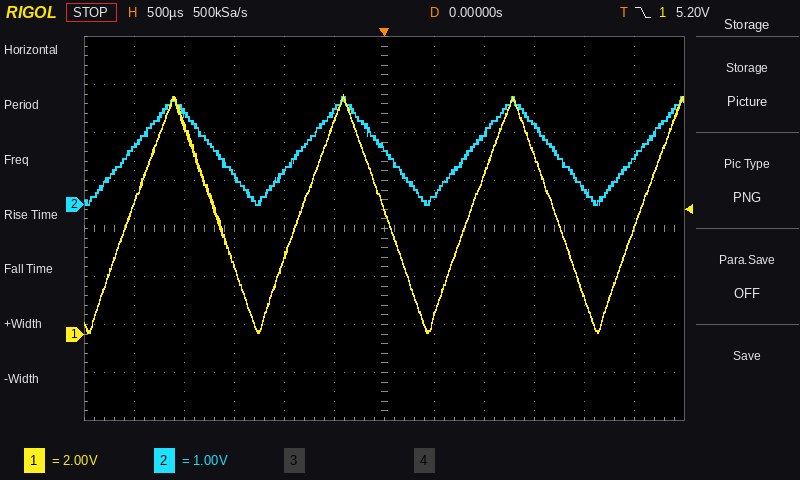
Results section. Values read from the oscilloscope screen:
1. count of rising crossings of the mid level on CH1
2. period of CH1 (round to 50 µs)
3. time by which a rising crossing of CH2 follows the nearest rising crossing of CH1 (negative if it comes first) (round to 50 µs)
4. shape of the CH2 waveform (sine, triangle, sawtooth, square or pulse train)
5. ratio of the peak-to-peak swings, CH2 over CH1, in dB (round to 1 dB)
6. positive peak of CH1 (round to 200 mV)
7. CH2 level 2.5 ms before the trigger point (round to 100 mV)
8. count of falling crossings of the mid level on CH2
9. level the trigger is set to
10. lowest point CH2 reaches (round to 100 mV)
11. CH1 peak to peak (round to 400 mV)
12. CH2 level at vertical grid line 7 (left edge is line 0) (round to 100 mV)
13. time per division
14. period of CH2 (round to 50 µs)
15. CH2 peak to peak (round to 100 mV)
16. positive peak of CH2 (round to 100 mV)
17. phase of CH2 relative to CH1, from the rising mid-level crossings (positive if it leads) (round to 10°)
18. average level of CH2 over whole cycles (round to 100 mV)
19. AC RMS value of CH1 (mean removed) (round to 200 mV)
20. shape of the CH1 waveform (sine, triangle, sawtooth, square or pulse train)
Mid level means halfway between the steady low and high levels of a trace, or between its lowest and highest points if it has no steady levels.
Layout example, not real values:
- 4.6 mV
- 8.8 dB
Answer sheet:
- 4
- 1.70 ms
- 0 µs
- triangle
- -13 dB
- 10.0 V
- 1.2 V
- 3
- 5.20 V
- 0.0 V
- 10.0 V
- 200 mV
- 500 µs
- 1.70 ms
- 2.2 V
- 2.2 V
- 0°
- 1.1 V
- 2.8 V
- triangle
